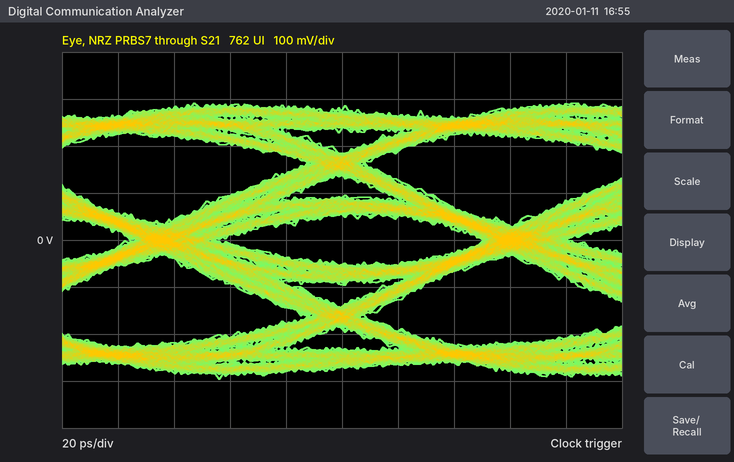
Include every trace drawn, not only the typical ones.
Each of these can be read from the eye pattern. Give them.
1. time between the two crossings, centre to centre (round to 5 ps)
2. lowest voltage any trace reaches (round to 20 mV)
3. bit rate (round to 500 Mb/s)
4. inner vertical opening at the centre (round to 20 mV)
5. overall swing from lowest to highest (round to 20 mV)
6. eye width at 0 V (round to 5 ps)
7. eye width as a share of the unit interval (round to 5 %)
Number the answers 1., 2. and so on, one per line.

1. 125 ps
2. -300 mV
3. 8.0 Gb/s
4. 100 mV
5. 580 mV
6. 95 ps
7. 75 %
